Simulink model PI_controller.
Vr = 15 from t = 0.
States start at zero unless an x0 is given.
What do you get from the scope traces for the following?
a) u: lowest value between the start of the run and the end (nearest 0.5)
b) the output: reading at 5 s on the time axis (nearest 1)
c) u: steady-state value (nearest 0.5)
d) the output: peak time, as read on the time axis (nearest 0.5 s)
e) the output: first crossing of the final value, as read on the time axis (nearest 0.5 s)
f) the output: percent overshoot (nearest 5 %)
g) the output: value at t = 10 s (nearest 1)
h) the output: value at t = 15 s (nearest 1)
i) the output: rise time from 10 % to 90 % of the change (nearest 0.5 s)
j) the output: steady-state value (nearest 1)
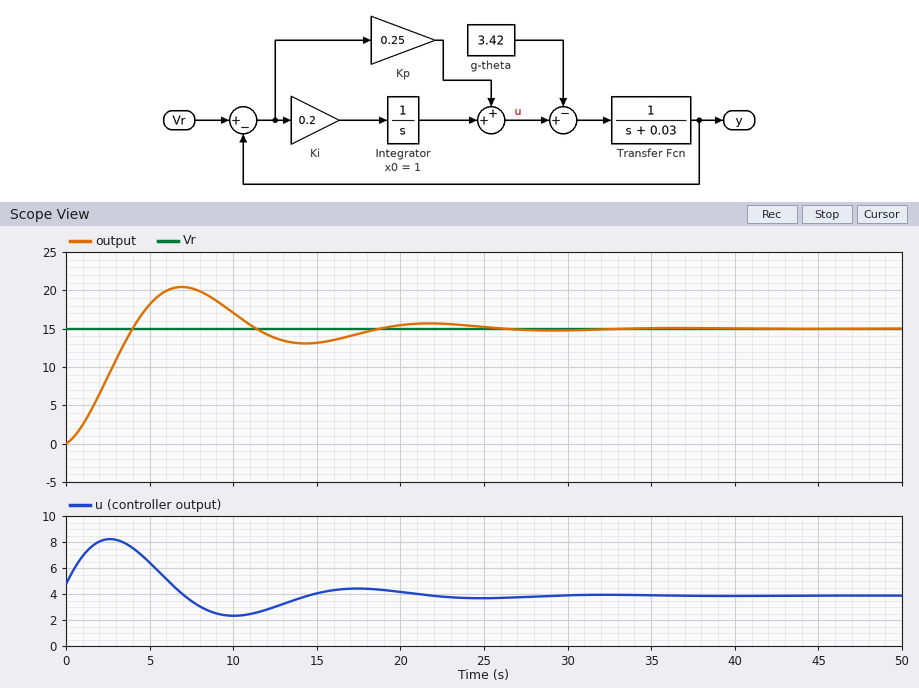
2.5
18
4.0
7.0 s
4.0 s
35 %
17
13
3.0 s
15
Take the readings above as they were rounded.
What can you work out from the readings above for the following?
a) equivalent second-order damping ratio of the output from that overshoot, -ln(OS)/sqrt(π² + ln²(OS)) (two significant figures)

0.32
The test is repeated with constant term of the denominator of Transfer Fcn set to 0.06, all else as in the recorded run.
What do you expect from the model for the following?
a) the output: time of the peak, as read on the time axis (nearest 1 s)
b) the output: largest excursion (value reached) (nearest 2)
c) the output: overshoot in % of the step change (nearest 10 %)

7 s
20
30 %
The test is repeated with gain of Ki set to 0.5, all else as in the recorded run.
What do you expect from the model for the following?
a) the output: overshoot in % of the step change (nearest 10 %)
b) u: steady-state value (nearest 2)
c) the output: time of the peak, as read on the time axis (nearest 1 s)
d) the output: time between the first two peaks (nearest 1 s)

50 %
4
4 s
9 s
